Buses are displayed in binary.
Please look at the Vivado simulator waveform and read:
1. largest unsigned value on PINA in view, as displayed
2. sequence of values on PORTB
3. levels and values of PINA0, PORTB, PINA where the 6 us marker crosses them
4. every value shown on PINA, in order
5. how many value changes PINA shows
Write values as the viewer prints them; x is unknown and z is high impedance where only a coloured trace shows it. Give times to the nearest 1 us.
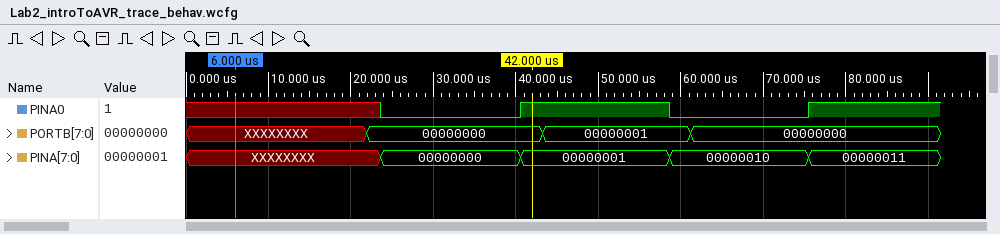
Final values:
00000011
XXXXXXXX, 00000000, 00000001, 00000000
PINA0=x, PORTB=XXXXXXXX, PINA=XXXXXXXX
XXXXXXXX, 00000000, 00000001, 00000010, 00000011
4
